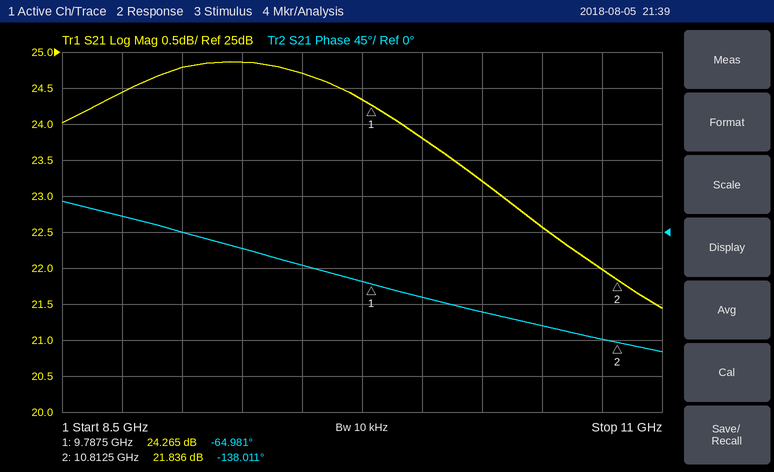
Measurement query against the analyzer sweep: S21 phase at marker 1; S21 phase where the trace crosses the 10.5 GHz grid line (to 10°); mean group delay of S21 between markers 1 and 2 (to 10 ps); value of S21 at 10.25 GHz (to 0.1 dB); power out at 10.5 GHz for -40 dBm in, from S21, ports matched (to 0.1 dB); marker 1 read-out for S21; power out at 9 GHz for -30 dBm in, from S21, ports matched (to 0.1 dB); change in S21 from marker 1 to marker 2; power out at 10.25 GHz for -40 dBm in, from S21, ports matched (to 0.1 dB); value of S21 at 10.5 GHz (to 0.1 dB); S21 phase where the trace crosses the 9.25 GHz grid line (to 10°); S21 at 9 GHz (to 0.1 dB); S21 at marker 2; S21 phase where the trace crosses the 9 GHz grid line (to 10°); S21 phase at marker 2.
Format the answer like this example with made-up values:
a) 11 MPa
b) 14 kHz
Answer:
a) -64.981°
b) -120°
c) 200 ps
d) 23.2 dB
e) -17.4 dBm
f) 24.265 dB
g) -5.2 dBm
h) -2.429 dB
i) -16.8 dBm
j) 22.6 dB
k) -20°
l) 24.8 dB
m) 21.836 dB
n) 0°
o) -138.011°
